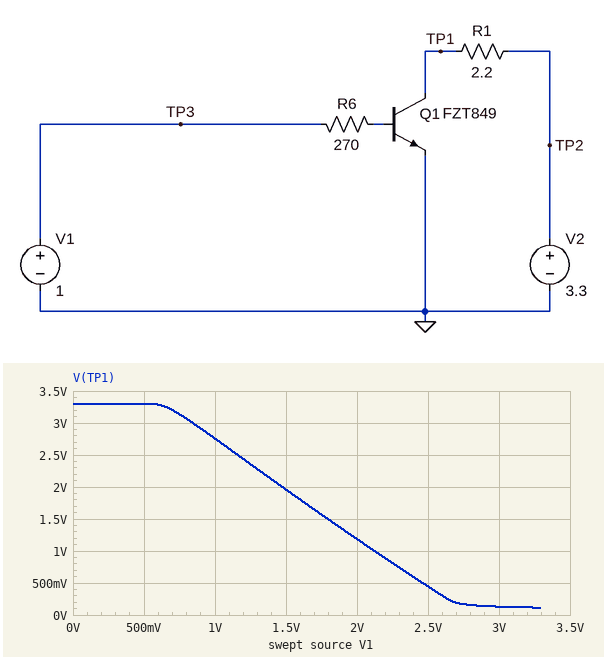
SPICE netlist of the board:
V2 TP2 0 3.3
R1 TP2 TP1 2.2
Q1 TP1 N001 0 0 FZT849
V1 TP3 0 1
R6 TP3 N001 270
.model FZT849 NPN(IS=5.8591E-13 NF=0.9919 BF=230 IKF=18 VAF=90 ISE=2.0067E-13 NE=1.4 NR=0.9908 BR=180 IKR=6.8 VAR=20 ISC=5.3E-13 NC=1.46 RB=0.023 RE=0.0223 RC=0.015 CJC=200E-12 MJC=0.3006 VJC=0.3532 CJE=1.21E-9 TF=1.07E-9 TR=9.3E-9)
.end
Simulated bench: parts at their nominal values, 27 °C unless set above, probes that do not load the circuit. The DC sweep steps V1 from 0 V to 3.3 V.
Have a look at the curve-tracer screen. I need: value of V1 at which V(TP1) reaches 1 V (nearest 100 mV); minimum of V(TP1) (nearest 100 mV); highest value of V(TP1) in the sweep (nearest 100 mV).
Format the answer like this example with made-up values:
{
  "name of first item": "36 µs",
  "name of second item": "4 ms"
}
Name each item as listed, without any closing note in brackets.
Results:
{
  "value of V1 at which V(TP1) reaches 1 V": "2.1 V",
  "minimum of V(TP1)": "100 mV",
  "highest value of V(TP1) in the sweep": "3.3 V"
}
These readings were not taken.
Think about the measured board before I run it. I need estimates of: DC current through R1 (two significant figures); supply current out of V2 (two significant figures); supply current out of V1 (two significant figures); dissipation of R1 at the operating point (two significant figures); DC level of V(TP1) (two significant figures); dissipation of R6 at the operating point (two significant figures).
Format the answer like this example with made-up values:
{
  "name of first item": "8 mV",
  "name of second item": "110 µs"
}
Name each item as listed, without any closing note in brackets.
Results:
{
  "DC current through R1": "250 mA",
  "supply current out of V2": "250 mA",
  "supply current out of V1": "1.1 mA",
  "dissipation of R1 at the operating point": "130 mW",
  "DC level of V(TP1)": "2.8 V",
  "dissipation of R6 at the operating point": "350 µW"
}
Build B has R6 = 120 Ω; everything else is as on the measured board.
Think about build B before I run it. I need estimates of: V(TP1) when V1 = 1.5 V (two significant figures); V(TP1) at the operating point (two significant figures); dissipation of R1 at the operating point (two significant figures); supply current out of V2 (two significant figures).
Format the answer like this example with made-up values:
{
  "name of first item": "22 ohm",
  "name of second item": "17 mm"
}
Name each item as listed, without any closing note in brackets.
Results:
{
  "V(TP1) when V1 = 1.5 V": "550 mV",
  "V(TP1) at the operating point": "2.2 V",
  "dissipation of R1 at the operating point": "560 mW",
  "supply current out of V2": "500 mA"
}
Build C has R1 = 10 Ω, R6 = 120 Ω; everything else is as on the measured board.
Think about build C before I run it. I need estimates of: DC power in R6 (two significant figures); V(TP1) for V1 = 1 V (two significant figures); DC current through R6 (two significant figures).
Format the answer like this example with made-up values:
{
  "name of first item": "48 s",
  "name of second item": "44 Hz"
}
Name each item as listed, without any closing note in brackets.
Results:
{
  "DC power in R6": "710 µW",
  "V(TP1) for V1 = 1 V": "55 mV",
  "DC current through R6": "2.4 mA"
}
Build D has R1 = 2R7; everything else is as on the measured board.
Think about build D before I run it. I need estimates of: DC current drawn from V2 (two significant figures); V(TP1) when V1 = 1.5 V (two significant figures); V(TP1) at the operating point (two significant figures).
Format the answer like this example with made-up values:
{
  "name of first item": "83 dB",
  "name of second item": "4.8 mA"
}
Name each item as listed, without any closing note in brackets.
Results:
{
  "DC current drawn from V2": "250 mA",
  "V(TP1) when V1 = 1.5 V": "1.7 V",
  "V(TP1) at the operating point": "2.6 V"
}
